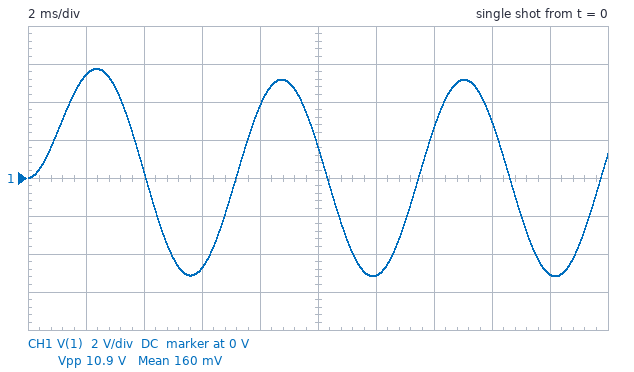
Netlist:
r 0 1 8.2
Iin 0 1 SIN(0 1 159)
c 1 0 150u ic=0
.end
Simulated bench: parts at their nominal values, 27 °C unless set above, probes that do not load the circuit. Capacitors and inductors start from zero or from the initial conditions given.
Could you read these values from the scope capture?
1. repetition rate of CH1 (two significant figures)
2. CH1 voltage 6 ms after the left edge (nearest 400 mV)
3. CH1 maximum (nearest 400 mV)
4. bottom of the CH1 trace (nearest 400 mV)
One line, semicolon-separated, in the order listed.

160 Hz; -4.8 V; 5.6 V; -5.2 V
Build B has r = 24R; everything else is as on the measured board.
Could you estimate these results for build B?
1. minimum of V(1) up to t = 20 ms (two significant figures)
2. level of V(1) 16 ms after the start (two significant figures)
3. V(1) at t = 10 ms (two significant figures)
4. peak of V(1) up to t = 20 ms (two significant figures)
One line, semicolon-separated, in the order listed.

-6.4 V; 5.6 V; 4.7 V; 9.3 V
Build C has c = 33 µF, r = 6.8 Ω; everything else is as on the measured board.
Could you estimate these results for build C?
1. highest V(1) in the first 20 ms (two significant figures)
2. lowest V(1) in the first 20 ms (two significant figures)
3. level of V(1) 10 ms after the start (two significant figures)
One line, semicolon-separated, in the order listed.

6.6 V; -6.6 V; -2.2 V
